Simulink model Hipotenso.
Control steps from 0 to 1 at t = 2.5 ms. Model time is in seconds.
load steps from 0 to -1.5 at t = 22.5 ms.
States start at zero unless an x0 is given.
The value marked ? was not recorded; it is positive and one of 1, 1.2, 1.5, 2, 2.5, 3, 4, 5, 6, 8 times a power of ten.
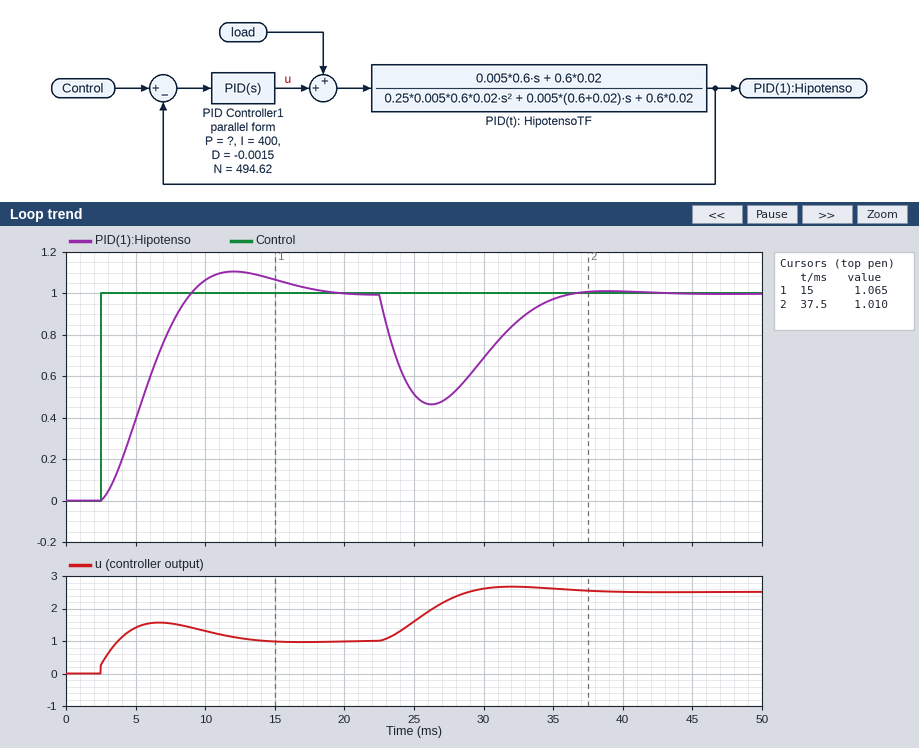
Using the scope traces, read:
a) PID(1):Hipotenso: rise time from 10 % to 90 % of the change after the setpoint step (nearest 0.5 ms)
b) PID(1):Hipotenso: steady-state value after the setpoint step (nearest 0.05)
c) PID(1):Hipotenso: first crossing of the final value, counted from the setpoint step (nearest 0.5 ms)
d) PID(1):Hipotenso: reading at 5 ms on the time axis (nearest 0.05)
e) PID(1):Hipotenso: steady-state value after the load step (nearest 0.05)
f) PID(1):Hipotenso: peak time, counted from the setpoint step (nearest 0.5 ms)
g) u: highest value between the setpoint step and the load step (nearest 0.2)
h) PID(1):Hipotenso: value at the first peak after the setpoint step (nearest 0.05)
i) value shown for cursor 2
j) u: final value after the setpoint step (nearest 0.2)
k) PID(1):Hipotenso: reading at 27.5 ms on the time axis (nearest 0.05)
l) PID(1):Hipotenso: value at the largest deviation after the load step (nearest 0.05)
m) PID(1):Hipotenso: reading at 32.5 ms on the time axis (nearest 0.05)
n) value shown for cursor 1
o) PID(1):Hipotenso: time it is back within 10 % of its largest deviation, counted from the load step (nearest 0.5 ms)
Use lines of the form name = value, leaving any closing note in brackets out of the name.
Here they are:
PID(1):Hipotenso: rise time from 10 % to 90 % of the change after the setpoint step = 4.5 ms
PID(1):Hipotenso: steady-state value after the setpoint step = 1.00
PID(1):Hipotenso: first crossing of the final value, counted from the setpoint step = 6.5 ms
PID(1):Hipotenso: reading at 5 ms on the time axis = 0.40
PID(1):Hipotenso: steady-state value after the load step = 1.00
PID(1):Hipotenso: peak time, counted from the setpoint step = 9.5 ms
u: highest value between the setpoint step and the load step = 1.6
PID(1):Hipotenso: value at the first peak after the setpoint step = 1.10
value shown for cursor 2 = 1.010
u: final value after the setpoint step = 1.0
PID(1):Hipotenso: reading at 27.5 ms on the time axis = 0.50
PID(1):Hipotenso: value at the largest deviation after the load step = 0.45
PID(1):Hipotenso: reading at 32.5 ms on the time axis = 0.85
value shown for cursor 1 = 1.065
PID(1):Hipotenso: time it is back within 10 % of its largest deviation, counted from the load step = 11.5 ms
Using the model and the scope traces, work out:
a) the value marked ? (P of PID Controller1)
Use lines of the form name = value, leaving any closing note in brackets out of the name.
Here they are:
the value marked ? = 1
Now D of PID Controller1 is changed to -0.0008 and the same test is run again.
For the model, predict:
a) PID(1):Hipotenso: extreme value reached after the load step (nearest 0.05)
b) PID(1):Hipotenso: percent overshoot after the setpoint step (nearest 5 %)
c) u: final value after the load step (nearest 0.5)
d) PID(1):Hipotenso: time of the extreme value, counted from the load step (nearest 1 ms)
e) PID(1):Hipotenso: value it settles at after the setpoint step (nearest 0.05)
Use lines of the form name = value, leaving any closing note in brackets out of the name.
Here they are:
PID(1):Hipotenso: extreme value reached after the load step = 0.50
PID(1):Hipotenso: percent overshoot after the setpoint step = 10 %
u: final value after the load step = 2.5
PID(1):Hipotenso: time of the extreme value, counted from the load step = 4 ms
PID(1):Hipotenso: value it settles at after the setpoint step = 1.00
